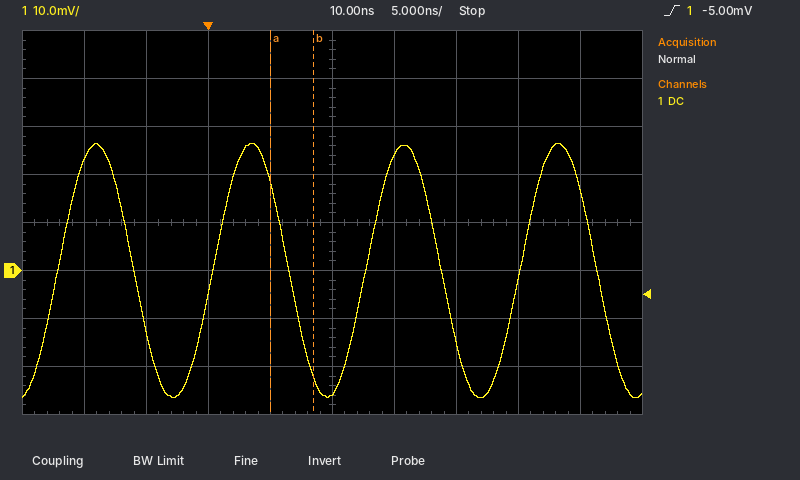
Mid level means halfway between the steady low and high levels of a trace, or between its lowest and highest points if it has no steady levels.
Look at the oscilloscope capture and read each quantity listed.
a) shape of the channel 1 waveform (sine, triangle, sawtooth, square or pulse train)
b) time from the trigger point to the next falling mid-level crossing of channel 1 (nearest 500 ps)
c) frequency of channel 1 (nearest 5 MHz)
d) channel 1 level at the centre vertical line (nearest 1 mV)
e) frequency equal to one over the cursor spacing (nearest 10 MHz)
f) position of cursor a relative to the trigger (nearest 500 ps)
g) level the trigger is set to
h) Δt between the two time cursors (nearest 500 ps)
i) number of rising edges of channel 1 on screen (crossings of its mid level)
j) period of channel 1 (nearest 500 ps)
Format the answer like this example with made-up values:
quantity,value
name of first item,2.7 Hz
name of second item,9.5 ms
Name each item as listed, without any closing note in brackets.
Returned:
quantity,value
shape of the channel 1 waveform,sine
time from the trigger point to the next falling mid-level crossing of channel 1,6.5 ns
frequency of channel 1,80 MHz
channel 1 level at the centre vertical line,-26 mV
frequency equal to one over the cursor spacing,290 MHz
position of cursor a relative to the trigger,+5.0 ns
level the trigger is set to,-5.00 mV
Δt between the two time cursors,3.5 ns
number of rising edges of channel 1 on screen,4
period of channel 1,12.5 ns
